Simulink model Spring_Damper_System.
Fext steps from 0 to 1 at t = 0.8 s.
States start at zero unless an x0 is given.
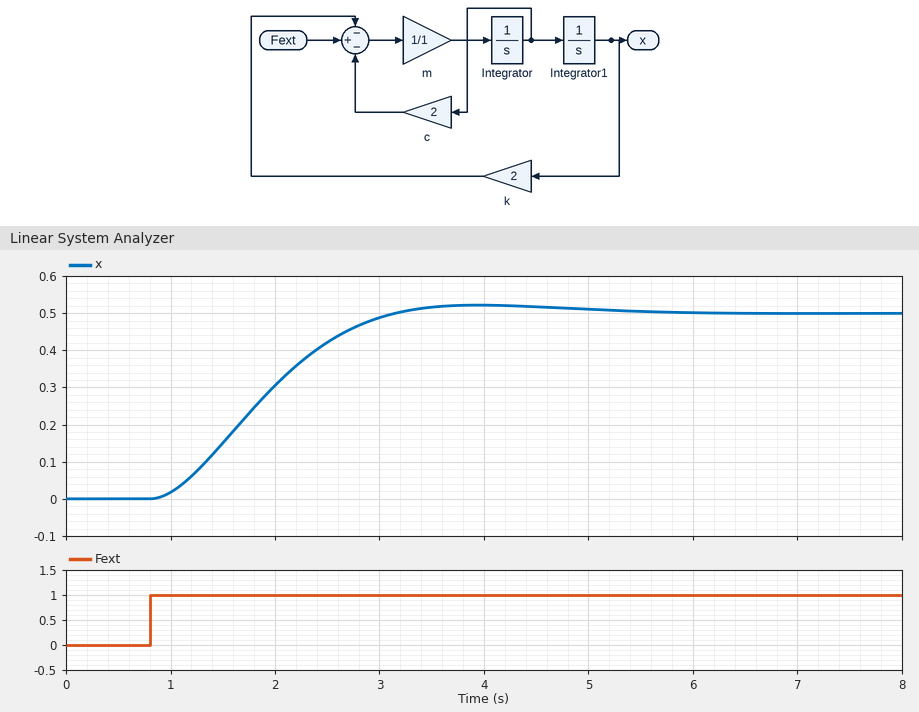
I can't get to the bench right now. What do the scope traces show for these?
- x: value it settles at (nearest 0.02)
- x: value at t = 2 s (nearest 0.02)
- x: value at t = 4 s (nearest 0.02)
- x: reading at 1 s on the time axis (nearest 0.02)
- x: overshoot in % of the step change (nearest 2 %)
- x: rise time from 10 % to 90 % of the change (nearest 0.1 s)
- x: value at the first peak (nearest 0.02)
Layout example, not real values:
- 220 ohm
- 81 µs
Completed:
- 0.50
- 0.30
- 0.52
- 0.02
- 4 %
- 1.5 s
- 0.52
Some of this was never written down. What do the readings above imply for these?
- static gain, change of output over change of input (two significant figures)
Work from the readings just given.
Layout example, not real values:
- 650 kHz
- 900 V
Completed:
- 0.50
